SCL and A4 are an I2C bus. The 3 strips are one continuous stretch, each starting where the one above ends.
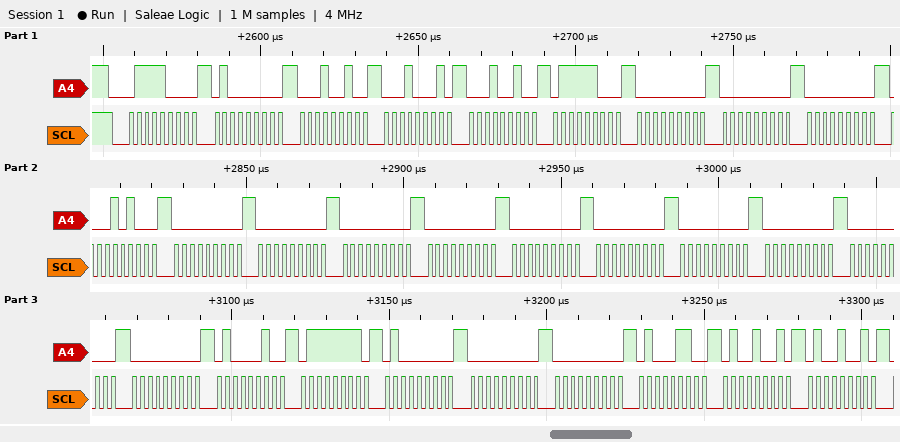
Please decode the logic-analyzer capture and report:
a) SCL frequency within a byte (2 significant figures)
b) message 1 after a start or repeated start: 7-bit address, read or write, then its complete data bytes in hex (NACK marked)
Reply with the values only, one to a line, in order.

400 kHz
0x3C write: 40 12 11 12 7C 00 00 00 14 00 00 00 00 00 00 00 00 00 00 42 7F 40 00 00 46 49 49
